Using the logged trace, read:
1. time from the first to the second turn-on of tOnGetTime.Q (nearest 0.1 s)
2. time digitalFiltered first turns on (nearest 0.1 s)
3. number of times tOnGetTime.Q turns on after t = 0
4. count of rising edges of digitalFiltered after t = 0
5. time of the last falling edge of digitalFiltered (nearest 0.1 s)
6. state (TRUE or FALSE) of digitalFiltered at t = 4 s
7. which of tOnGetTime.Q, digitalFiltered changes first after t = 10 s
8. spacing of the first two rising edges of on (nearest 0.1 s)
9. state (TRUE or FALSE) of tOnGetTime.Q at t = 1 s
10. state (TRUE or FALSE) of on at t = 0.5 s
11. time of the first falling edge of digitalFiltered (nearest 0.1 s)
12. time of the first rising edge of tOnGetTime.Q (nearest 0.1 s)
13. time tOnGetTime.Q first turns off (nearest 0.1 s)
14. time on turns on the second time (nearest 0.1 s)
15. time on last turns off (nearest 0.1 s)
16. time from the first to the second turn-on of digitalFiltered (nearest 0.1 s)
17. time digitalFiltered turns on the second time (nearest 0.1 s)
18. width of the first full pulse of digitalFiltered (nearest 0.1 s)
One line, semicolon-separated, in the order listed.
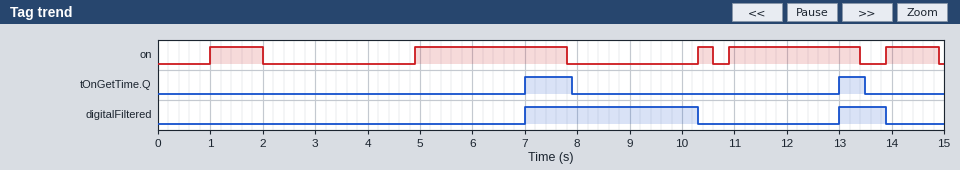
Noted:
6.0 s; 7.0 s; 2; 2; 13.9 s; FALSE; digitalFiltered; 3.9 s; FALSE; FALSE; 10.3 s; 7.0 s; 7.9 s; 4.9 s; 14.9 s; 6.0 s; 13.0 s; 3.3 s
